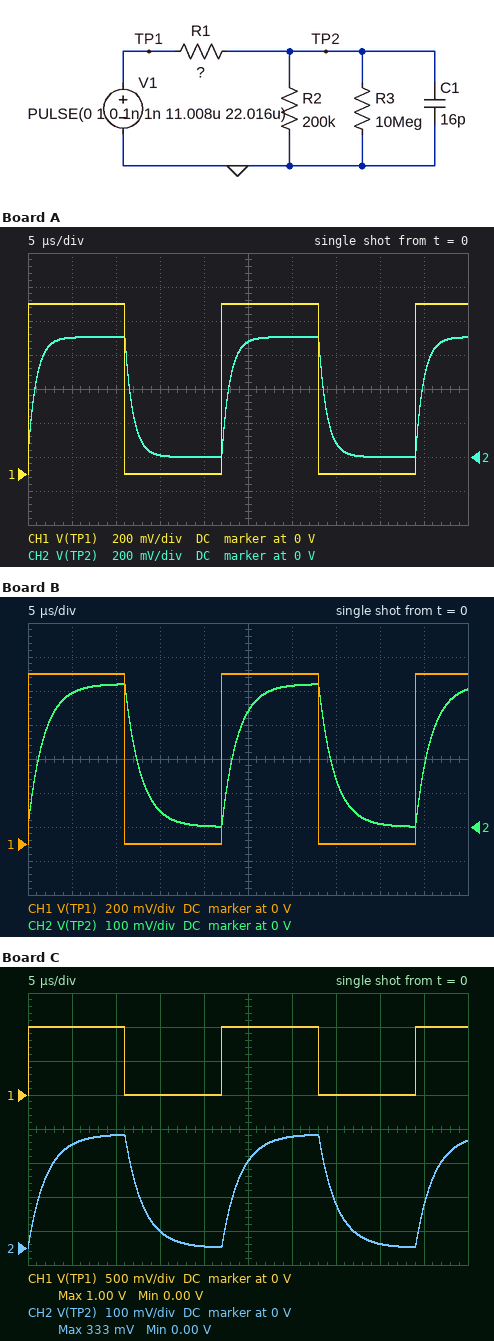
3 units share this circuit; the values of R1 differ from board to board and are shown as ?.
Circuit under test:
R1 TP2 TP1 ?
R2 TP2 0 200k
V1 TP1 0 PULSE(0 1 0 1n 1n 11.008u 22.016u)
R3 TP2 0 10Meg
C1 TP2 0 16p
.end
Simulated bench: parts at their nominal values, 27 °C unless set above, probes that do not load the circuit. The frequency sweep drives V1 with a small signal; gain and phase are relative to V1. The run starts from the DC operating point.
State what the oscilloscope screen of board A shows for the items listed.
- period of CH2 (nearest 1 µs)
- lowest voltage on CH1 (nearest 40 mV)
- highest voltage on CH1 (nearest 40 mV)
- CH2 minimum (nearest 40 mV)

22 µs
0 V
1.00 V
0 V
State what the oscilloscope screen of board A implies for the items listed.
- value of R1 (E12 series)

82 kΩ
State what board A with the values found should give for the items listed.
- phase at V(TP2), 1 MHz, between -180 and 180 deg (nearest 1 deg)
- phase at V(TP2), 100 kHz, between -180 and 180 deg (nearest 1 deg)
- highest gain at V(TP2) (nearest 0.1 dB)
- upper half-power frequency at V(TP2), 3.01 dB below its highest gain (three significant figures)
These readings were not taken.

-80 deg
-30 deg
-3.0 dB
172 kHz
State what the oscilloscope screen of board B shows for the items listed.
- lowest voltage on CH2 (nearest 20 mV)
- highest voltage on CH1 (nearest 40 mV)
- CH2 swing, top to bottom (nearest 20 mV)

0 V
1.00 V
420 mV
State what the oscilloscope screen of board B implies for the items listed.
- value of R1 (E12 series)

270 kΩ
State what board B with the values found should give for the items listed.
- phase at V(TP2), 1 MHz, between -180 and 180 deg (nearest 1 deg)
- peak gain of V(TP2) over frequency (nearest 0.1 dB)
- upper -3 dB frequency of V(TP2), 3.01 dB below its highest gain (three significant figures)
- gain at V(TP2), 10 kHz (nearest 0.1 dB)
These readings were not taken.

-85 deg
-7.5 dB
87.6 kHz
-7.6 dB
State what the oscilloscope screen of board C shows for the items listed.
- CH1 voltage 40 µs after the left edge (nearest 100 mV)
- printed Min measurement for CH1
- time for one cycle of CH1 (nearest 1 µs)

0 V
0.00 V
22 µs
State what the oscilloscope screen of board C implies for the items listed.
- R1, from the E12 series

390 kΩ
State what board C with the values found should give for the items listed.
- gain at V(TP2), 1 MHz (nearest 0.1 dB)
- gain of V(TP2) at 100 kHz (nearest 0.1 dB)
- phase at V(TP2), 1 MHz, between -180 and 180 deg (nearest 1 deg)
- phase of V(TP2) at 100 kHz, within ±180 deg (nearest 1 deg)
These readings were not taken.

-31.9 dB
-13.9 dB
-86 deg
-53 deg
